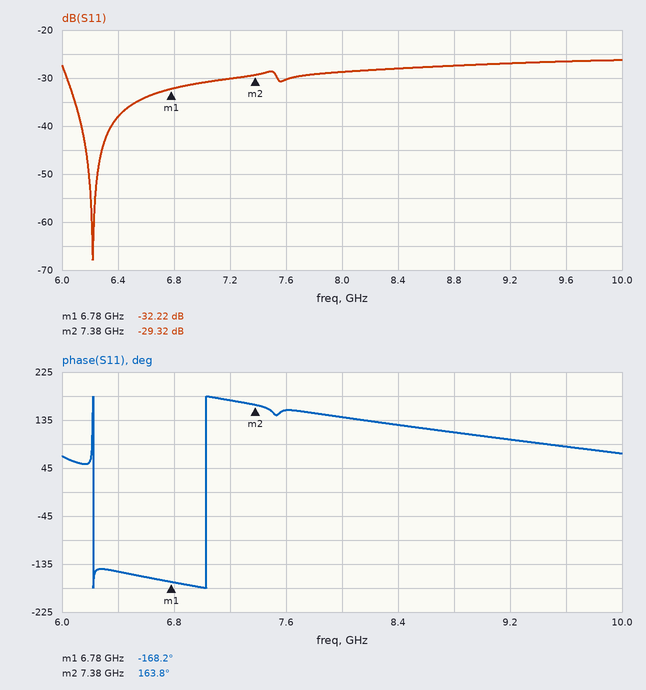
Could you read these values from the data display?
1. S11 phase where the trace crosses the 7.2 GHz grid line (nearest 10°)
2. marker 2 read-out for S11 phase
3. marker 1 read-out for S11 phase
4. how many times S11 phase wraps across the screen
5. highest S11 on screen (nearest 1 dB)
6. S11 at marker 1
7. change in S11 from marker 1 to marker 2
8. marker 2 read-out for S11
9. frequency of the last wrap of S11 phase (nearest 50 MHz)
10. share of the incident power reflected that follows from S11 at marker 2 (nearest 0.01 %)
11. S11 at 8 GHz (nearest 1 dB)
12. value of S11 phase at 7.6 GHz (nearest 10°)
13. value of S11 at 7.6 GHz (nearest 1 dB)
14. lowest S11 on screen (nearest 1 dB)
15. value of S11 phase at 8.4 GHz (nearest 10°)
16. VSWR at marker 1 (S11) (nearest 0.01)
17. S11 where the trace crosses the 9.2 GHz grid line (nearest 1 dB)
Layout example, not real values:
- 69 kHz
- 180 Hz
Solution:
- 170°
- 163.8°
- -168.2°
- 2
- -26 dB
- -32.22 dB
- 2.90 dB
- -29.32 dB
- 7.05 GHz
- 0.12 %
- -29 dB
- 150°
- -30 dB
- -68 dB
- 130°
- 1.05
- -27 dB
